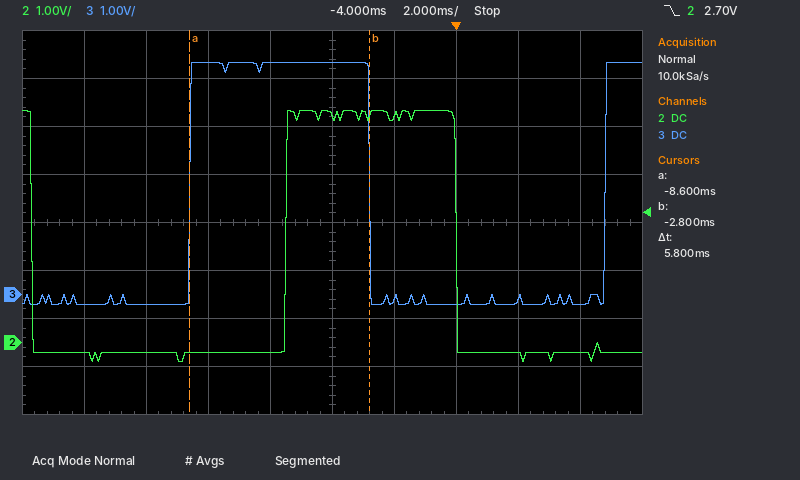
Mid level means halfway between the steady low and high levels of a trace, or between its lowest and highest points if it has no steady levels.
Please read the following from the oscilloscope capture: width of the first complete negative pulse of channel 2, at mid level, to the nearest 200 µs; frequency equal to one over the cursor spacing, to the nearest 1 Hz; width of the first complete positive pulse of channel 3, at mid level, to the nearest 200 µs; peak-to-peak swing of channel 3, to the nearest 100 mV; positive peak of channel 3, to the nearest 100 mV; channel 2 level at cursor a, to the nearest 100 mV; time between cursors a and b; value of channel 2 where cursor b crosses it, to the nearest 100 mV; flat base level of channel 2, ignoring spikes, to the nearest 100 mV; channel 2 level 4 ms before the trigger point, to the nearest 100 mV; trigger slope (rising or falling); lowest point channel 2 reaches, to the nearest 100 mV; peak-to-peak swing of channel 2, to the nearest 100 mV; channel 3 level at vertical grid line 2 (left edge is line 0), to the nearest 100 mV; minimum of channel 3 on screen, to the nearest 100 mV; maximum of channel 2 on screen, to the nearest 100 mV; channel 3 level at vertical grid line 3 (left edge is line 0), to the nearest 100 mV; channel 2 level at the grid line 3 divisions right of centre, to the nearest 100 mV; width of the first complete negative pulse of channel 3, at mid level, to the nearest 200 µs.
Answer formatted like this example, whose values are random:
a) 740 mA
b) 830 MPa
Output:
a) 8.2 ms
b) 172 Hz
c) 5.8 ms
d) 5.0 V
e) 4.8 V
f) -200 mV
g) 5.8 ms
h) 4.7 V
i) -200 mV
j) 4.7 V
k) falling
l) -400 mV
m) 5.2 V
n) -200 mV
o) -200 mV
p) 4.8 V
q) 4.8 V
r) -200 mV
s) 7.6 ms
